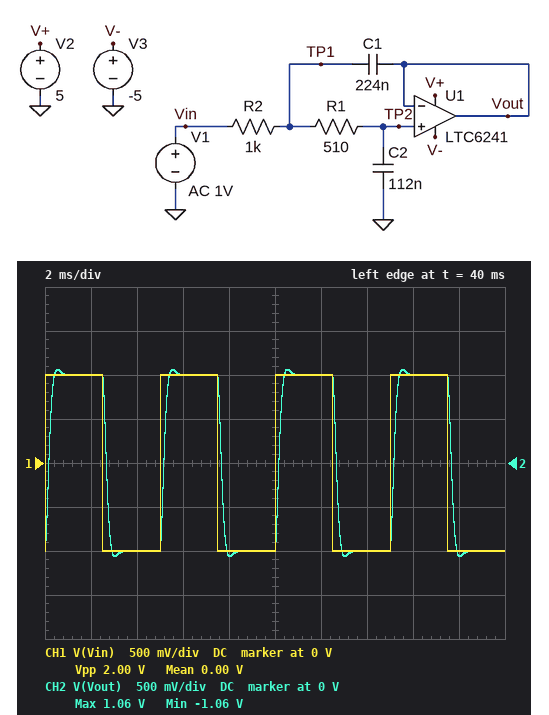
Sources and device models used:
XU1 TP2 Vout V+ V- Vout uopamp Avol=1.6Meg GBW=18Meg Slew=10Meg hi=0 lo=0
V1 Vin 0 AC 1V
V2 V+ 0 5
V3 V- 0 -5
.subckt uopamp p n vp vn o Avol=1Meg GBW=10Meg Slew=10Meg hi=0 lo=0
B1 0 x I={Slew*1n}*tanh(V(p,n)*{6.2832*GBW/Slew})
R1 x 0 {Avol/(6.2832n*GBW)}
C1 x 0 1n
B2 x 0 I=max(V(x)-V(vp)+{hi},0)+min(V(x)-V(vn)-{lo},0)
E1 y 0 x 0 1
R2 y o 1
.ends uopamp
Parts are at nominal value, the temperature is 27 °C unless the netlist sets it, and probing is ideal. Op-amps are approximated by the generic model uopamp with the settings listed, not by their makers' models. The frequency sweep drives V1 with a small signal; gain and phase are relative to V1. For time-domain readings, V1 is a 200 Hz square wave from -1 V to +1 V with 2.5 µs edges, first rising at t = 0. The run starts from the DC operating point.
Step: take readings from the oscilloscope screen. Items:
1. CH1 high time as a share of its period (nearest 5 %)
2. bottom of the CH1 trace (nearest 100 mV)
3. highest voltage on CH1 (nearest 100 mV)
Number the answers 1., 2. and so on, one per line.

1. 50 %
2. -1.0 V
3. 1.0 V
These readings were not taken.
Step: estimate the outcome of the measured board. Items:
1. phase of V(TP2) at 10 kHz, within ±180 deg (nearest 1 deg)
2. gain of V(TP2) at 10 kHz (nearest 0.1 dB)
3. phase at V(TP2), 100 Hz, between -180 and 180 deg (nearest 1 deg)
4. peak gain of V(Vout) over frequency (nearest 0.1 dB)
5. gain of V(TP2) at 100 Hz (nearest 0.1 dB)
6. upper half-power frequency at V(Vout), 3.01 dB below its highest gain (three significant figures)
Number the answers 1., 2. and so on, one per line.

1. -168 deg
2. -34.1 dB
3. -6 deg
4. 0 dB
5. 0 dB
6. 1.33 kHz
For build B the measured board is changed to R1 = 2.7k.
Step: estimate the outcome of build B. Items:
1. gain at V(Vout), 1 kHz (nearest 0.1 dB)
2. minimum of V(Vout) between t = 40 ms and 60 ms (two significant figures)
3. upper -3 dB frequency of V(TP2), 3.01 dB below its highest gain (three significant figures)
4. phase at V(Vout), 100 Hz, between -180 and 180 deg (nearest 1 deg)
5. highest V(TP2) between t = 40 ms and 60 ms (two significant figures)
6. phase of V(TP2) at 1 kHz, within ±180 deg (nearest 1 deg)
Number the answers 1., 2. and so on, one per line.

1. -9.8 dB
2. -1.0 V
3. 536 Hz
4. -15 deg
5. 1.0 V
6. -123 deg
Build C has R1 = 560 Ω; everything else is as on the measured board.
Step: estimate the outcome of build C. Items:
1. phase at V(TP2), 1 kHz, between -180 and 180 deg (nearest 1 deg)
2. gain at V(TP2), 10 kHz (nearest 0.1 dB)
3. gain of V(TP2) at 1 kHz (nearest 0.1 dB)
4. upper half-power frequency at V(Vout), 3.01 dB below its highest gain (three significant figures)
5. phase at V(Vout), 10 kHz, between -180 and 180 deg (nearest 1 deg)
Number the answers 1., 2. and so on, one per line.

1. -68 deg
2. -34.9 dB
3. -1.5 dB
4. 1.29 kHz
5. -169 deg
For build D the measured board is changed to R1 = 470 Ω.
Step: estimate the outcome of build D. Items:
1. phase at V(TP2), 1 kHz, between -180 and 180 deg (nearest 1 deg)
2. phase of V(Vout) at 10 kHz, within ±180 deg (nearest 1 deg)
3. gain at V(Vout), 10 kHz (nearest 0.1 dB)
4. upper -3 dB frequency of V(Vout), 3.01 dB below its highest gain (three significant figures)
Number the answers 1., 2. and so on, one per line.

1. -63 deg
2. -167 deg
3. -33.4 dB
4. 1.36 kHz
